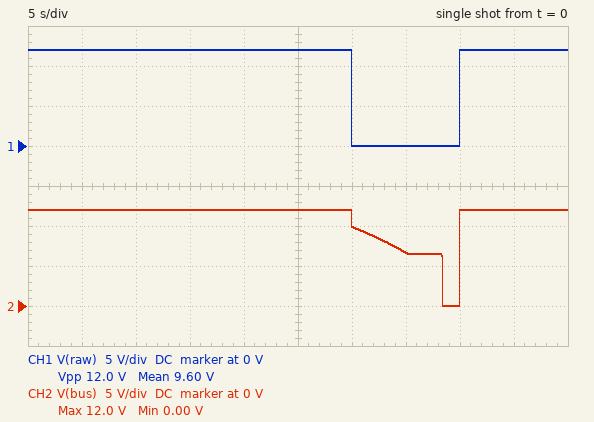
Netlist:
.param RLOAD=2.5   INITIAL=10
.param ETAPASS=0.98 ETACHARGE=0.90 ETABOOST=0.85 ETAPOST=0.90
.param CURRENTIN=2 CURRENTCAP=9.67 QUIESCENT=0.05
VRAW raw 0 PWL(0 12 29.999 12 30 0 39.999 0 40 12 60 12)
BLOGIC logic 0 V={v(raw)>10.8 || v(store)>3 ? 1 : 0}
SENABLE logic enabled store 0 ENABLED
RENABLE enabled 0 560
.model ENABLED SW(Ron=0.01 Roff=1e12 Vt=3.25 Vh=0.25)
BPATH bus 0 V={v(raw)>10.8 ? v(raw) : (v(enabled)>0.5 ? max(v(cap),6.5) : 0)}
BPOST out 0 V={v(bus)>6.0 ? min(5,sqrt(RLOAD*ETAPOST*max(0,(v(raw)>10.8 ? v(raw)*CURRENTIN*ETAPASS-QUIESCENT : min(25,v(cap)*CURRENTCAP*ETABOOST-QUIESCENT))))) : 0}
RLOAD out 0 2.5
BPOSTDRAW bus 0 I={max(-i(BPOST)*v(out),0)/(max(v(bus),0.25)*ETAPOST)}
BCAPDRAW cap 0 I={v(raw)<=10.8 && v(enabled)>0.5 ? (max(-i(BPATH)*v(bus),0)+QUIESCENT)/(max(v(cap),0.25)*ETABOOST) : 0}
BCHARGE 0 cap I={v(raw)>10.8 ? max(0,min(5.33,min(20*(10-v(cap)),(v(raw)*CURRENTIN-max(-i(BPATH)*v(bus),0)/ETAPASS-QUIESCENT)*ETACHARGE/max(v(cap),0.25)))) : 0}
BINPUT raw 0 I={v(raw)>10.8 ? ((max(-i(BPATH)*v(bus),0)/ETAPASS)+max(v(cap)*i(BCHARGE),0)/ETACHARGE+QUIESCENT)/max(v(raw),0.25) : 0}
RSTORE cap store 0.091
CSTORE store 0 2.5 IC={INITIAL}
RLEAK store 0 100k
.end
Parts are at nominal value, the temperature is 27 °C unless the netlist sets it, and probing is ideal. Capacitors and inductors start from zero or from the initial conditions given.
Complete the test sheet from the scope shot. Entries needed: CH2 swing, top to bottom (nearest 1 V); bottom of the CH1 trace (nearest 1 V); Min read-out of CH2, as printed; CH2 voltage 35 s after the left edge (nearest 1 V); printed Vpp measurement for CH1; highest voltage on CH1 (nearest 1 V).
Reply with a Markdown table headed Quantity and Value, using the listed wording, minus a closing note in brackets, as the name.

| Quantity | Value |
|---|---|
| CH2 swing, top to bottom | 12 V |
| bottom of the CH1 trace | 0 V |
| Min read-out of CH2, as printed | 0.00 V |
| CH2 voltage 35 s after the left edge | 7 V |
| printed Vpp measurement for CH1 | 12.0 V |
| highest voltage on CH1 | 12 V |
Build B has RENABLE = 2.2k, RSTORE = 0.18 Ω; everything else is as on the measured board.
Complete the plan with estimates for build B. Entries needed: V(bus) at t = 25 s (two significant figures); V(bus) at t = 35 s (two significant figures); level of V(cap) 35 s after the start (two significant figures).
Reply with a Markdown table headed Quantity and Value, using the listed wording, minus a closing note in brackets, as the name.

| Quantity | Value |
|---|---|
| V(bus) at t = 25 s | 12 V |
| V(bus) at t = 35 s | 6.5 V |
| level of V(cap) 35 s after the start | 6.4 V |
